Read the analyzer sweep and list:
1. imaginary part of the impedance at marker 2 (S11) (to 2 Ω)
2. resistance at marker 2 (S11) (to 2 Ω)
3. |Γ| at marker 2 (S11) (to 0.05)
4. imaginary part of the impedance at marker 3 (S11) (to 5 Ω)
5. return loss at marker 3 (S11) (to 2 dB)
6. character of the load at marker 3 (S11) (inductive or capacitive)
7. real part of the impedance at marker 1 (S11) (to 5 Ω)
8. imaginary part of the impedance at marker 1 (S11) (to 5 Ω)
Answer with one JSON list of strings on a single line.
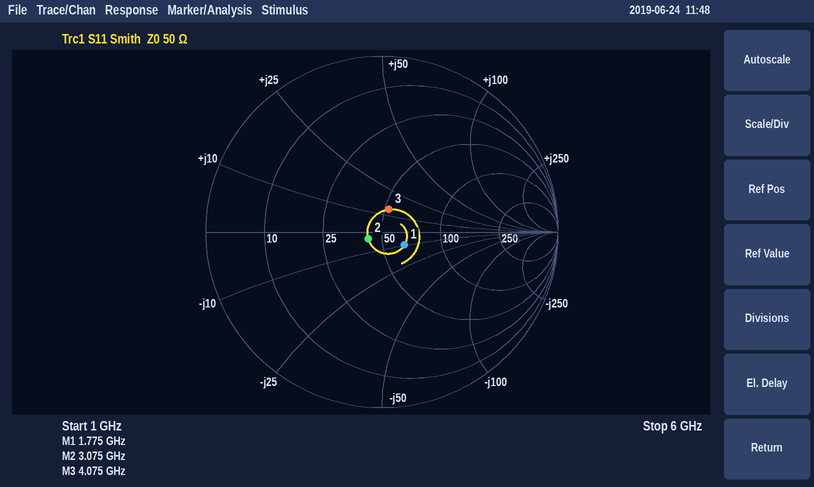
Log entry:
["-4 Ω", "42 Ω", "0.10", "+15 Ω", "18 dB", "inductive", "65 Ω", "-10 Ω"]
